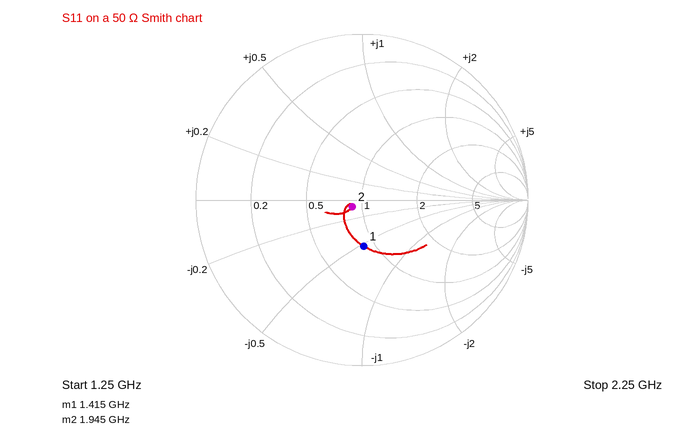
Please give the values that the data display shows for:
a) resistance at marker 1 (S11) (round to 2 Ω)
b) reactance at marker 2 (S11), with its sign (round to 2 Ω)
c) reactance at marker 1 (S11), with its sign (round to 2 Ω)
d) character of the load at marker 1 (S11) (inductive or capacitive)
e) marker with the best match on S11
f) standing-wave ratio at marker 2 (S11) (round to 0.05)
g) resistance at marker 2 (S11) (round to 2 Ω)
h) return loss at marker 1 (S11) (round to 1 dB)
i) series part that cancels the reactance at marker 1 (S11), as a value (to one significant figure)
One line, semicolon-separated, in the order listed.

44 Ω; -4 Ω; -26 Ω; capacitive; marker 2; 1.15; 44 Ω; 11 dB; 3 nH
